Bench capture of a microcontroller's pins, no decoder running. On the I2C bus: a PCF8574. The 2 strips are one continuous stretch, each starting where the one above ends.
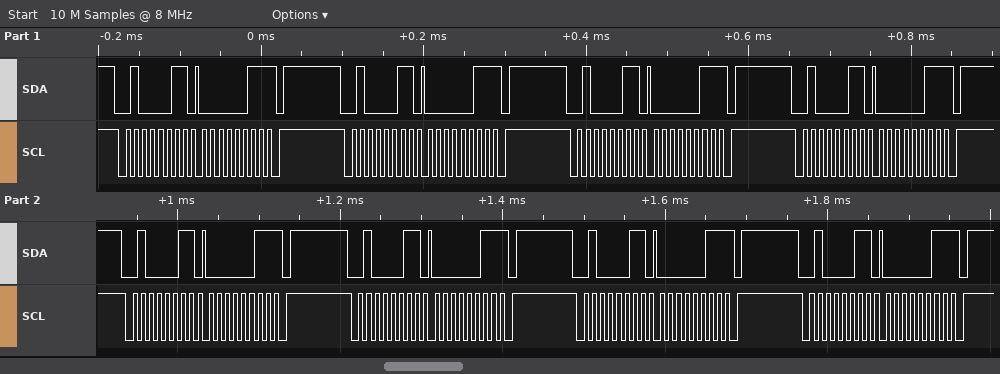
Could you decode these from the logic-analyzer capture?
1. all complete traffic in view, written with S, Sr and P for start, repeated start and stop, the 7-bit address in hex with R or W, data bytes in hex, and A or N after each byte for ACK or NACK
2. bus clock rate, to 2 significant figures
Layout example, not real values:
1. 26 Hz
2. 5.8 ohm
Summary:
1. S 21R A 03 N P S 21R A 03 N P S 21R A 03 N P S 21R A 03 N P S 21R A 03 N P S 21R A 03 N P S 21R A 03 N P S 21R A 03 N P
2. 100 kHz
